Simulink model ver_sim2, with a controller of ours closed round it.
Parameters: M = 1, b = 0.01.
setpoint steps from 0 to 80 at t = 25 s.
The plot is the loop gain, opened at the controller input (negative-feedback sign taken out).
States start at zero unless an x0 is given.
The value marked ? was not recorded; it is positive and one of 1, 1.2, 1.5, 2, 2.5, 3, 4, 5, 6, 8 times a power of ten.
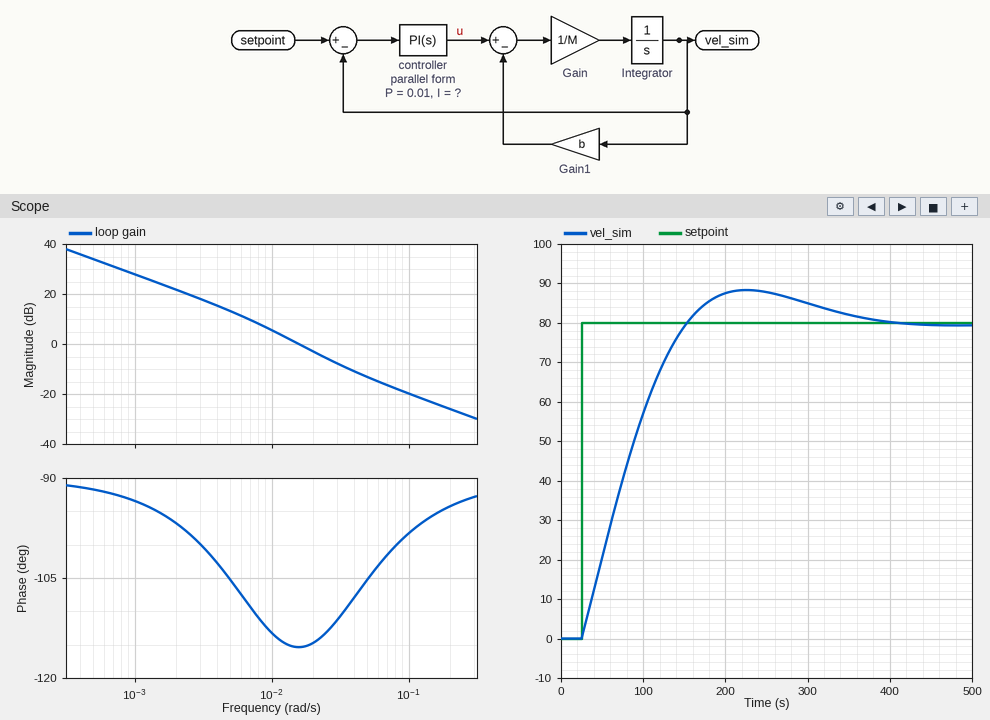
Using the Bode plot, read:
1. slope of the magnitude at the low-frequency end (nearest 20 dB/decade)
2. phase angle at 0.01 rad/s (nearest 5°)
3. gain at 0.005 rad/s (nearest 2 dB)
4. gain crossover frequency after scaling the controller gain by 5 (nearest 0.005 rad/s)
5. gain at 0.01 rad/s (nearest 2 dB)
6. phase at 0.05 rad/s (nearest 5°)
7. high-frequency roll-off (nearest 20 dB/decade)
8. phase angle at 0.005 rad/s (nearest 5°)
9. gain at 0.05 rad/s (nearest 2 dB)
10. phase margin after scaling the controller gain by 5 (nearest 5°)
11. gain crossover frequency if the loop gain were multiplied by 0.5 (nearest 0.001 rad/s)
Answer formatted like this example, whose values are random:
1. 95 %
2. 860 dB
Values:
1. -20 dB/decade
2. -115°
3. 14 dB
4. 0.055 rad/s
5. 6 dB
6. -105°
7. -20 dB/decade
8. -105°
9. -14 dB
10. 75°
11. 0.010 rad/s
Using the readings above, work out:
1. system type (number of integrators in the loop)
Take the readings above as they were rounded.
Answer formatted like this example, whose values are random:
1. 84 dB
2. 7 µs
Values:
1. 1
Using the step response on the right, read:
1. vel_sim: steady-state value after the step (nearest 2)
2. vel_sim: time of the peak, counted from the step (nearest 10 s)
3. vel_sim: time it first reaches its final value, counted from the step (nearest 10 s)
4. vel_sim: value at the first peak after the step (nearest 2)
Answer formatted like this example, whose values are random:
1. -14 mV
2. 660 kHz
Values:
1. 80
2. 200 s
3. 130 s
4. 88
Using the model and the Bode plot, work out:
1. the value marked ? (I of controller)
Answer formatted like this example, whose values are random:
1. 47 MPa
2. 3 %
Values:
1. 0.00025
